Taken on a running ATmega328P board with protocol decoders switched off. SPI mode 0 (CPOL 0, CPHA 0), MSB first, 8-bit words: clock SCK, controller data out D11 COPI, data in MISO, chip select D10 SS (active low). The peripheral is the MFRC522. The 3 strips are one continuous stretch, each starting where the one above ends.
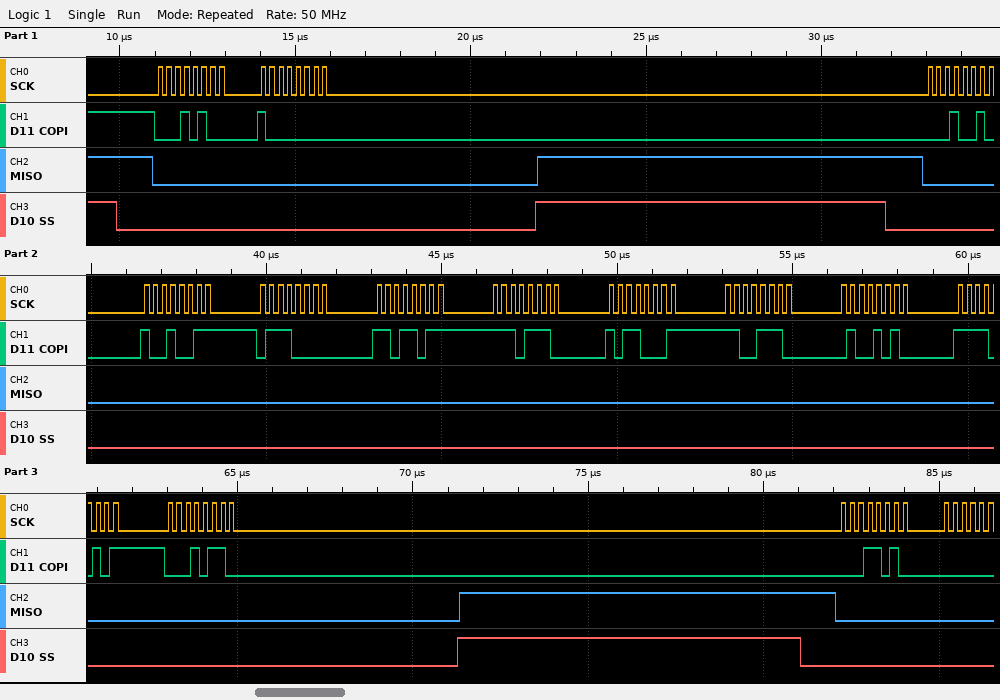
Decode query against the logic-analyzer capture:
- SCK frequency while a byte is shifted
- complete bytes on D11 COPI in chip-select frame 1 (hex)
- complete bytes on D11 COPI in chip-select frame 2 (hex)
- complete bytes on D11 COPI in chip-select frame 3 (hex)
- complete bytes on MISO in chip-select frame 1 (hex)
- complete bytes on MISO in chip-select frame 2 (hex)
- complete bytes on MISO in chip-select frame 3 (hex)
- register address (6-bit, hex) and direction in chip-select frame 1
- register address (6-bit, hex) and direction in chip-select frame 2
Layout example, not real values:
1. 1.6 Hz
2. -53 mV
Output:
1. 4 MHz
2. 0x14 0x80
3. 0x12 0x93 0x70 0xDB 0xEE 0xB1 0xCE 0x4A 0xF5 0x16
4. 0x1A
5. 0x00 0x00
6. 0x00 0x00 0x00 0x00 0x00 0x00 0x00 0x00 0x00 0x00
7. 0x00
8. 0x0A write
9. 0x09 write
